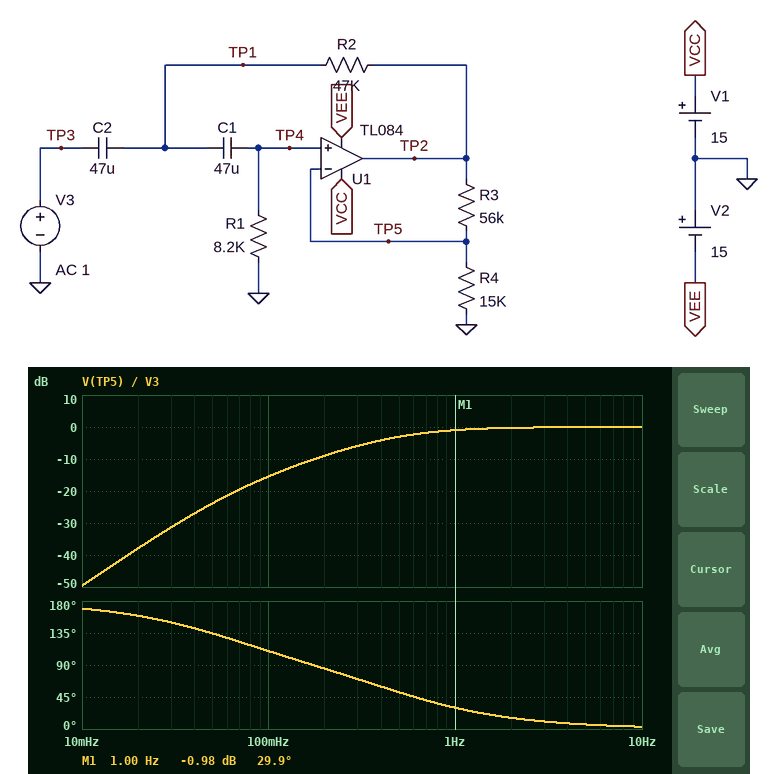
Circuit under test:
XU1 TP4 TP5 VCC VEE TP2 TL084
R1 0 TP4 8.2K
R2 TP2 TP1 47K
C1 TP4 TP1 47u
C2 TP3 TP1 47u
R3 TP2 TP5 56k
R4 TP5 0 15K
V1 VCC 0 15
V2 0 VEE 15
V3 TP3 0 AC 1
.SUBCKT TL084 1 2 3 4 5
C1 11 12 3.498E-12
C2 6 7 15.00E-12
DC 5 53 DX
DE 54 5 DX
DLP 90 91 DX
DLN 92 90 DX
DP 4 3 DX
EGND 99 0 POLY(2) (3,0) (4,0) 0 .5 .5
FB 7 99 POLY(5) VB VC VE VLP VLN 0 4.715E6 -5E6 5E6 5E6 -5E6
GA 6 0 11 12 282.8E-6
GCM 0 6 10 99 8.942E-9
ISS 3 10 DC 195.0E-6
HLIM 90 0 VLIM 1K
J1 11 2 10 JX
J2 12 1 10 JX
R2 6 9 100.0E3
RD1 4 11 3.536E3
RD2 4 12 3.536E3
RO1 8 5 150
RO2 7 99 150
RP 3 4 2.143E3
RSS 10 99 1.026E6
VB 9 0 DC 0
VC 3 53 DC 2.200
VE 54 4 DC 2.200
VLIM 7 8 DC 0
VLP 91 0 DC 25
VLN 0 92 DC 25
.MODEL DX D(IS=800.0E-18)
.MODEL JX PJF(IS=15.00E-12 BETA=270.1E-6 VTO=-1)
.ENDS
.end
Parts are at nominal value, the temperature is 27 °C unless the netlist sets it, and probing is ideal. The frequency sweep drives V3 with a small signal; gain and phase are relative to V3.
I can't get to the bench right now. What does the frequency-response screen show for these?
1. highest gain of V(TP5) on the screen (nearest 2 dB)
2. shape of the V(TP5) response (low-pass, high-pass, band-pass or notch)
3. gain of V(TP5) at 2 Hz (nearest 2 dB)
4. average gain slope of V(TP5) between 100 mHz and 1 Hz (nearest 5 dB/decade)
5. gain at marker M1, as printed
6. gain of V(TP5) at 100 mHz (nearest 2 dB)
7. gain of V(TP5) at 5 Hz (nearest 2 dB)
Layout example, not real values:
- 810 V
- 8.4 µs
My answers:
- 0 dB
- high-pass
- 0 dB
- 15 dB/decade
- -0.98 dB
- -16 dB
- 0 dB
